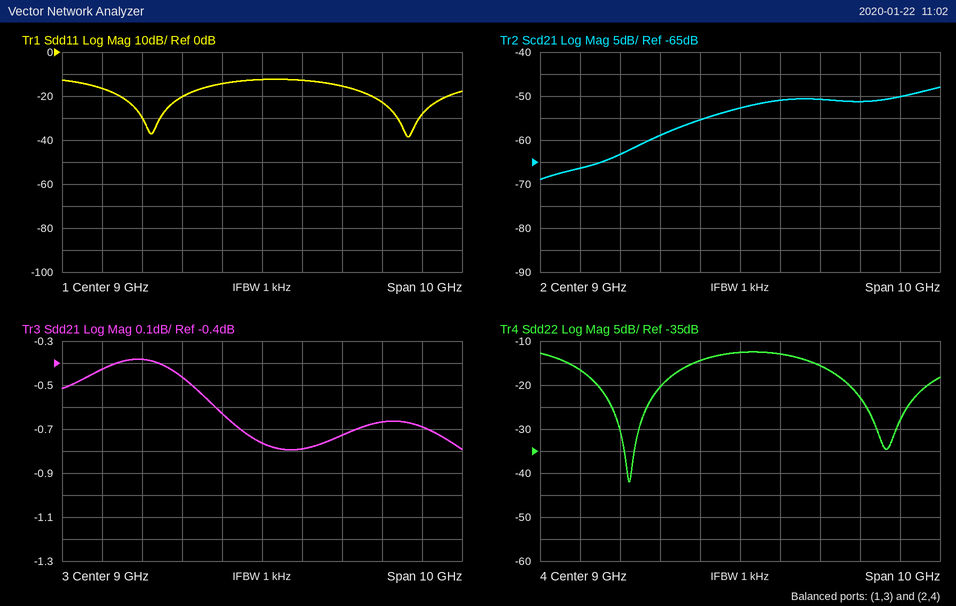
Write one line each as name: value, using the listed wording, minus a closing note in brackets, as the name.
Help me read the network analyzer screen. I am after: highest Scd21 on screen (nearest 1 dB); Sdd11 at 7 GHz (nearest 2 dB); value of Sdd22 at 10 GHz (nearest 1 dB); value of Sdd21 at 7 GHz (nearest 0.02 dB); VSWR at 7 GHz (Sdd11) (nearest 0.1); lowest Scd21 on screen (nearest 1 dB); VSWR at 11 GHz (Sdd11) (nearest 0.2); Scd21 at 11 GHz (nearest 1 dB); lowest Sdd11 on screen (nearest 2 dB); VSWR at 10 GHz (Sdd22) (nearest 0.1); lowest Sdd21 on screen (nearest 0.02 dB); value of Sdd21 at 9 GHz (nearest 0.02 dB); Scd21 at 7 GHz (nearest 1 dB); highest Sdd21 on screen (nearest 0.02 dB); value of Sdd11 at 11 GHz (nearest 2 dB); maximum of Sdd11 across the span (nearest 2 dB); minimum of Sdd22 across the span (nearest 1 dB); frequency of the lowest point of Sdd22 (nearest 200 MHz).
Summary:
highest Scd21 on screen: -48 dB
Sdd11 at 7 GHz: -20 dB
value of Sdd22 at 10 GHz: -13 dB
value of Sdd21 at 7 GHz: -0.46 dB
VSWR at 7 GHz (Sdd11): 1.2
lowest Scd21 on screen: -69 dB
VSWR at 11 GHz (Sdd11): 1.4
Scd21 at 11 GHz: -51 dB
lowest Sdd11 on screen: -38 dB
VSWR at 10 GHz (Sdd22): 1.6
lowest Sdd21 on screen: -0.80 dB
value of Sdd21 at 9 GHz: -0.76 dB
Scd21 at 7 GHz: -59 dB
highest Sdd21 on screen: -0.38 dB
value of Sdd11 at 11 GHz: -16 dB
maximum of Sdd11 across the span: -12 dB
minimum of Sdd22 across the span: -42 dB
frequency of the lowest point of Sdd22: 6.2 GHz
